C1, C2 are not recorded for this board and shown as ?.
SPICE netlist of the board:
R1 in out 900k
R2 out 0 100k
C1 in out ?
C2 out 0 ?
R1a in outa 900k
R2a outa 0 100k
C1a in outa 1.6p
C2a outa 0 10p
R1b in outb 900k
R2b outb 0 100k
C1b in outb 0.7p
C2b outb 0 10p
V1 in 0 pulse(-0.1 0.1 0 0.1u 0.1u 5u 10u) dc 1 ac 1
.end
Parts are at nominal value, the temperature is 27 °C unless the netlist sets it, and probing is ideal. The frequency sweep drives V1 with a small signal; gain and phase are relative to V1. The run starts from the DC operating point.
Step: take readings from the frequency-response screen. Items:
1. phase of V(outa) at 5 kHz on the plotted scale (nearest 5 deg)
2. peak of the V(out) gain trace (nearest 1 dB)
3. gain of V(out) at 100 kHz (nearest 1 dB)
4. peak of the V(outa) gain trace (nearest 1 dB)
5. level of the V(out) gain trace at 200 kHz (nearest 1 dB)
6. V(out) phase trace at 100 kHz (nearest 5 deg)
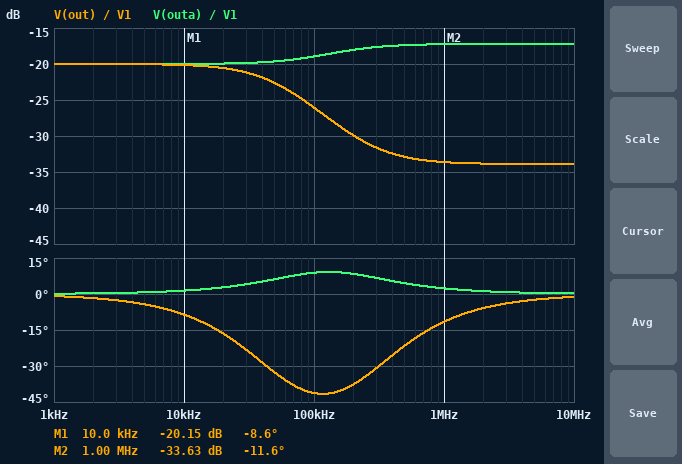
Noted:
0 deg
-20 dB
-26 dB
-17 dB
-30 dB
-40 deg
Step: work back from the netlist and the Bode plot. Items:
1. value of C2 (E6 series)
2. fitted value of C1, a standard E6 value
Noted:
33 pF
680 fF
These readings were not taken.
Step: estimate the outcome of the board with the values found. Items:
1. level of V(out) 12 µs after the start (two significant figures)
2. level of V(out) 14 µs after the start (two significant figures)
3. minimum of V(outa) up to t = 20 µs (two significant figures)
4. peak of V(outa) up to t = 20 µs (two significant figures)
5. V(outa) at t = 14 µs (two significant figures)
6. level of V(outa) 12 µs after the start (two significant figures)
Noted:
3.0 mV
6.4 mV
-17 mV
17 mV
10 mV
11 mV
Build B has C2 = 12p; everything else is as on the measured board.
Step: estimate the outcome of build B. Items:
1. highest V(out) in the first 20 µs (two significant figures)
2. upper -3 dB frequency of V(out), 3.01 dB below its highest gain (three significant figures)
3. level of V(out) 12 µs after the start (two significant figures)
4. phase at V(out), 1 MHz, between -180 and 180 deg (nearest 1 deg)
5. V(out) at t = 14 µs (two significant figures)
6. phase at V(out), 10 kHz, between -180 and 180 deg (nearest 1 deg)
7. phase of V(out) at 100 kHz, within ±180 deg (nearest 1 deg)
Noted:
9.9 mV
214 kHz
8.3 mV
-7 deg
9.7 mV
-2 deg
-15 deg
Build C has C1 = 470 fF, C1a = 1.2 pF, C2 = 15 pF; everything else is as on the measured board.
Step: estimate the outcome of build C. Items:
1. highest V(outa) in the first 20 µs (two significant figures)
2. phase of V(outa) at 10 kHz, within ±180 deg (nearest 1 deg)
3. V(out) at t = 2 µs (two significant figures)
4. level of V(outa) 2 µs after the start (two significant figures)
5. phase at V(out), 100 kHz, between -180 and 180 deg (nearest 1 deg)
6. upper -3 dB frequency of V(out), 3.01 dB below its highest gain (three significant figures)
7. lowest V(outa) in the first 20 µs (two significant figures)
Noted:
11 mV
0 deg
6.6 mV
10 mV
-26 deg
127 kHz
-11 mV
